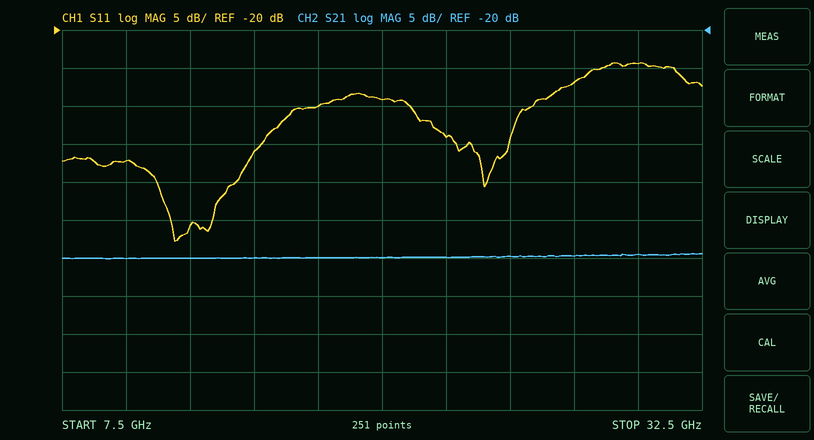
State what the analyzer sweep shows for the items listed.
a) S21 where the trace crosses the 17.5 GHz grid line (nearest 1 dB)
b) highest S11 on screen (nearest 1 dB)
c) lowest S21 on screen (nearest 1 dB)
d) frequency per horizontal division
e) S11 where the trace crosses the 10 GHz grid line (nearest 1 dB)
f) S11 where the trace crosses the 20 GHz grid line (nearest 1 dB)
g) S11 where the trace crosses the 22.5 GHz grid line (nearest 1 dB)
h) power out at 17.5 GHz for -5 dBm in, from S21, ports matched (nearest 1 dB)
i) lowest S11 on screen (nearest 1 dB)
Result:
-50 dB
-24 dB
-50 dB
2.5 GHz
-37 dB
-29 dB
-34 dB
-55 dBm
-48 dB
